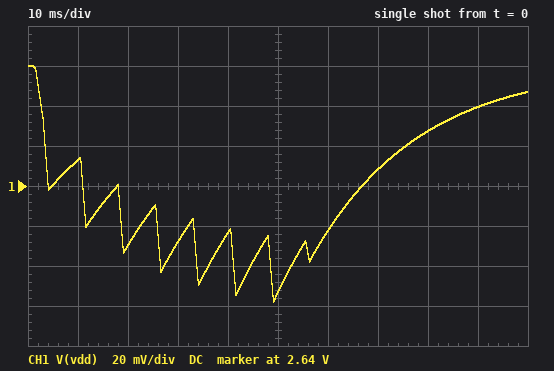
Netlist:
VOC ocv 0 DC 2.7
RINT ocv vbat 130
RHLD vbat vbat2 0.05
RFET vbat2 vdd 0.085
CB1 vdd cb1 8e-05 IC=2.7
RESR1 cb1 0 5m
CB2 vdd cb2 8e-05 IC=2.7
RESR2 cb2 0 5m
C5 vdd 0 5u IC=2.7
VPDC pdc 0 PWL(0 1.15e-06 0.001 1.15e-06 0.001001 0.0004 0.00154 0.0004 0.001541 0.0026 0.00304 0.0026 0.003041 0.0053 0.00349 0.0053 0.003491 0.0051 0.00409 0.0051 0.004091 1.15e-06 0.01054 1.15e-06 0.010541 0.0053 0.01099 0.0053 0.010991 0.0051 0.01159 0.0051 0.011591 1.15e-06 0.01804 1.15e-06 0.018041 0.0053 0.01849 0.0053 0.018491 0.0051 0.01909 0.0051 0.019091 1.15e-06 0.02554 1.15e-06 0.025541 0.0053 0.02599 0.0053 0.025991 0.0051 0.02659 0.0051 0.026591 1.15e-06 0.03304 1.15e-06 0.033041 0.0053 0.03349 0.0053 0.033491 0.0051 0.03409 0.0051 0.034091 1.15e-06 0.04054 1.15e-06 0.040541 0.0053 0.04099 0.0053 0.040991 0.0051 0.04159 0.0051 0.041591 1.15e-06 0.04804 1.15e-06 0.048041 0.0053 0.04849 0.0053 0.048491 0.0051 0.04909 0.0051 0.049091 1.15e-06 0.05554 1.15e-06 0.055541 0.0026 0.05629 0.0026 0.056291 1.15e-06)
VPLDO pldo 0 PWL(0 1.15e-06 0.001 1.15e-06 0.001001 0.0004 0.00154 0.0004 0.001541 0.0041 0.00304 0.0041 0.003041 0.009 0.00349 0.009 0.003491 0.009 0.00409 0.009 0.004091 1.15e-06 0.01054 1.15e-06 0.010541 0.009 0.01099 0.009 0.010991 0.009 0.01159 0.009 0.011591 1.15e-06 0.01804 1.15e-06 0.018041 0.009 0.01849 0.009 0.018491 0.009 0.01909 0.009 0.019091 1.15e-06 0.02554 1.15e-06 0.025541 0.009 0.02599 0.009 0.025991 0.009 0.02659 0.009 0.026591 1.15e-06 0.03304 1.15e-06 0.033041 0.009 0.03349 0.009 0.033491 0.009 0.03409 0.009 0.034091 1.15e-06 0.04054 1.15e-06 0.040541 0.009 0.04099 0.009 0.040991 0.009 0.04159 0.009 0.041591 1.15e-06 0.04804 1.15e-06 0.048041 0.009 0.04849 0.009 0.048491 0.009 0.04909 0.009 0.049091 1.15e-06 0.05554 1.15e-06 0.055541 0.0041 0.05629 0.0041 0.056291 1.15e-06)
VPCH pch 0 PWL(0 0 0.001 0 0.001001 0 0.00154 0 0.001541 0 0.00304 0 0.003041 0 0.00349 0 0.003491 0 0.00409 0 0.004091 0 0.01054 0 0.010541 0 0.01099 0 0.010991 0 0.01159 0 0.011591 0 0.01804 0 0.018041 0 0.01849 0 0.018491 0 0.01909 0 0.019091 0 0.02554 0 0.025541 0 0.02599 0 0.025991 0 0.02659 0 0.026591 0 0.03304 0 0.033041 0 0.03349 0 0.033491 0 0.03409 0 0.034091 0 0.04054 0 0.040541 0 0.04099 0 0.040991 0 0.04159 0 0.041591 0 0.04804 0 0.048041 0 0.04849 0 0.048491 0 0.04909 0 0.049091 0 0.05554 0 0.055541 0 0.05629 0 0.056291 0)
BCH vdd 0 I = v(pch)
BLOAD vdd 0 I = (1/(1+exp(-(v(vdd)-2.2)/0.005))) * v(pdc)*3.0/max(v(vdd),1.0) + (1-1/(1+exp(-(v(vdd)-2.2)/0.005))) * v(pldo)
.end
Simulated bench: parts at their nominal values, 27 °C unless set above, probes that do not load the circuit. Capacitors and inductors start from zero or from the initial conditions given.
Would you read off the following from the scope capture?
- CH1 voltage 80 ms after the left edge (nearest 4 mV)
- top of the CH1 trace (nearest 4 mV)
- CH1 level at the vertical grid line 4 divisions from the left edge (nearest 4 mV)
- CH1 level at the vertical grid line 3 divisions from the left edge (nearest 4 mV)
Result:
2.668 V
2.700 V
2.616 V
2.612 V
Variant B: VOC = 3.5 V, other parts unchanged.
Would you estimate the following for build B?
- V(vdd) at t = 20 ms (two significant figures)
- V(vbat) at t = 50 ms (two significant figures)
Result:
3.1 V
3.3 V
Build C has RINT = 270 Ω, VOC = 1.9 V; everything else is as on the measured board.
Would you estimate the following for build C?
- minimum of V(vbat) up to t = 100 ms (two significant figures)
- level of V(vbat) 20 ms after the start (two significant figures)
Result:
1.9 V
2.3 V
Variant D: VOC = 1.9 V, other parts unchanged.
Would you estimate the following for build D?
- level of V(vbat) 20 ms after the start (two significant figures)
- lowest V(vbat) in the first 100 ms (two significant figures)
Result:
2.1 V
1.8 V
